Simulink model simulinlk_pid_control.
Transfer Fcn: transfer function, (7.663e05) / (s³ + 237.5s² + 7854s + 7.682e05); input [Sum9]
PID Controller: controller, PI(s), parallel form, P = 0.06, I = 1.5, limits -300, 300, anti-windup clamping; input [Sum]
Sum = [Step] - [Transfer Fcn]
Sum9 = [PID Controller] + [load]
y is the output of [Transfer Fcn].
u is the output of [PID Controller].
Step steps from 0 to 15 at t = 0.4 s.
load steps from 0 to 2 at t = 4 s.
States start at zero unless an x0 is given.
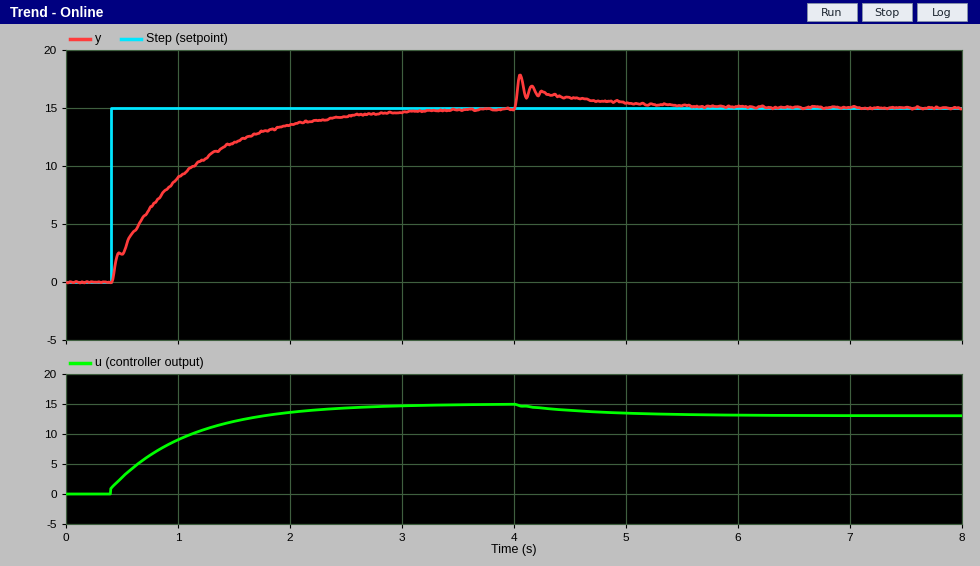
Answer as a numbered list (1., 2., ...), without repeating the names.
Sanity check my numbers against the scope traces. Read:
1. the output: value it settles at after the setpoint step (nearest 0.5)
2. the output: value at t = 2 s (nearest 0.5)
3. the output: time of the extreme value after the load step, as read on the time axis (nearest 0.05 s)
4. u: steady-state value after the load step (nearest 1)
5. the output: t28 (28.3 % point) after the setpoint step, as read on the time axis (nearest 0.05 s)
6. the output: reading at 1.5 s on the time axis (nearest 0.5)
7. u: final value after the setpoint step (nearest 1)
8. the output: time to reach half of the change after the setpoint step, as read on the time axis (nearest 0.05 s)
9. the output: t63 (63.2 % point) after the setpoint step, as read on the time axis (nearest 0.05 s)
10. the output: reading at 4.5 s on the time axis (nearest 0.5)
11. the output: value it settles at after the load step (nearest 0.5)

1. 15.0
2. 13.5
3. 4.05 s
4. 13
5. 0.60 s
6. 12.0
7. 15
8. 0.85 s
9. 1.05 s
10. 16.0
11. 15.0
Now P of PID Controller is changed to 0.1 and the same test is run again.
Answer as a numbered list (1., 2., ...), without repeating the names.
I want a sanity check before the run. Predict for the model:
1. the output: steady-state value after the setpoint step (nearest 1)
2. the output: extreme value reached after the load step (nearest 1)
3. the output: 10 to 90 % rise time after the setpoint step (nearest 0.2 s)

1. 15
2. 18
3. 1.6 s
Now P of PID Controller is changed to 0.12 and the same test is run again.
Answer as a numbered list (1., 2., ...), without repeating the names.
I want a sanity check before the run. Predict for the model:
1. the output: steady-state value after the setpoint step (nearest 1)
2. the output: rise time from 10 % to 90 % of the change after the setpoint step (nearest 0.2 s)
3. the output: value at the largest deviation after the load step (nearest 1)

1. 15
2. 1.6 s
3. 18
